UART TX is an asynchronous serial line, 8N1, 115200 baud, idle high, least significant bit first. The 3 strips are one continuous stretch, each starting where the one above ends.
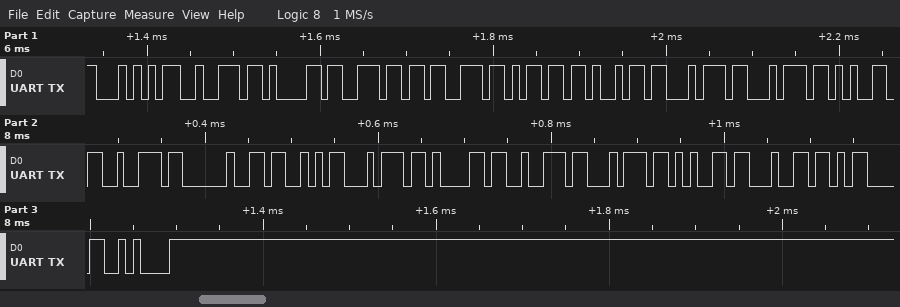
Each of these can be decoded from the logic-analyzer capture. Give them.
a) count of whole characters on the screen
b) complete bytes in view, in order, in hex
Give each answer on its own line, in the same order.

21
54 72 61 6E 73 6D 69 74 74 65 72 20 53 74 61 72 74 65 64 0D 0A
